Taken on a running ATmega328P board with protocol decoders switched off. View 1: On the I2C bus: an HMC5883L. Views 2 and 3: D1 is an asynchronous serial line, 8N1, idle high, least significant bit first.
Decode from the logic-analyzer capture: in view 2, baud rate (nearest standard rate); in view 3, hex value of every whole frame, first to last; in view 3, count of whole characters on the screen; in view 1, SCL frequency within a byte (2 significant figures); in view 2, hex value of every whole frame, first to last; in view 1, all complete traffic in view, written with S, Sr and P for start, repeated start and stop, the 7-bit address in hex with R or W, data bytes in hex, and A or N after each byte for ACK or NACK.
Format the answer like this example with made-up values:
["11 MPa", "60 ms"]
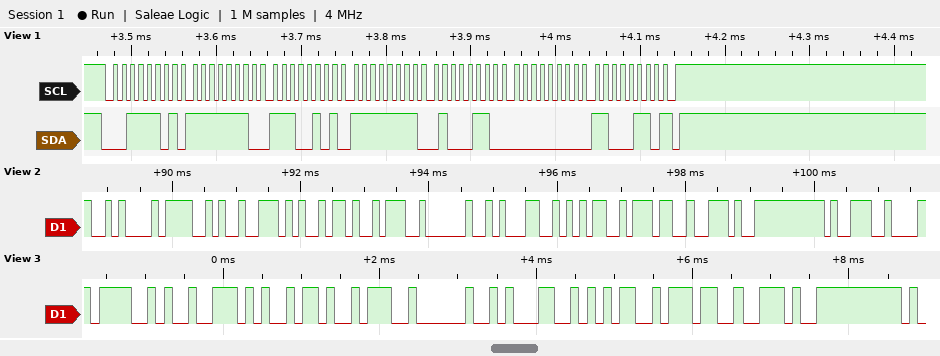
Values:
["9600 baud", "0x4F 0x72 0x69 0x3A 0x20 0x31 0x35 0x37 0x2E", "9", "100 kHz", "0A 4F 72 69 3A 20 31 35 37 2E 39", "S 1ER A FE A E5 A FF A 46 A 00 A C6 N P"]
